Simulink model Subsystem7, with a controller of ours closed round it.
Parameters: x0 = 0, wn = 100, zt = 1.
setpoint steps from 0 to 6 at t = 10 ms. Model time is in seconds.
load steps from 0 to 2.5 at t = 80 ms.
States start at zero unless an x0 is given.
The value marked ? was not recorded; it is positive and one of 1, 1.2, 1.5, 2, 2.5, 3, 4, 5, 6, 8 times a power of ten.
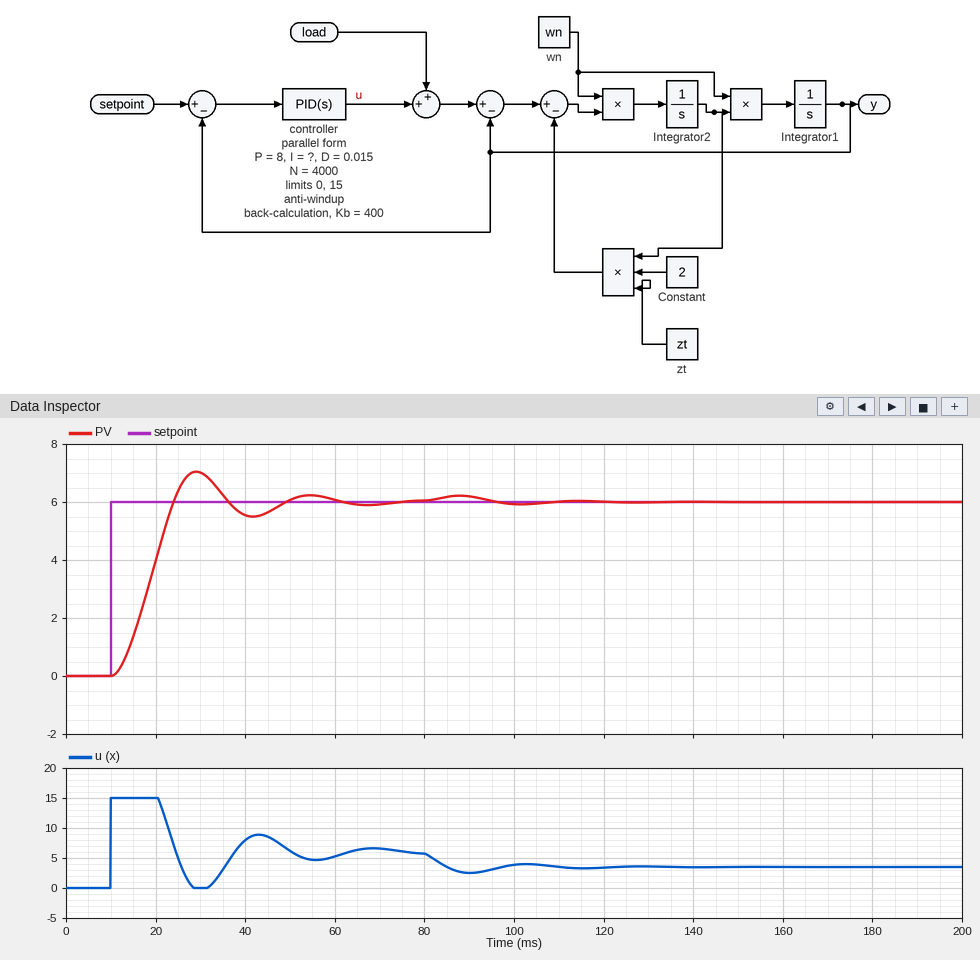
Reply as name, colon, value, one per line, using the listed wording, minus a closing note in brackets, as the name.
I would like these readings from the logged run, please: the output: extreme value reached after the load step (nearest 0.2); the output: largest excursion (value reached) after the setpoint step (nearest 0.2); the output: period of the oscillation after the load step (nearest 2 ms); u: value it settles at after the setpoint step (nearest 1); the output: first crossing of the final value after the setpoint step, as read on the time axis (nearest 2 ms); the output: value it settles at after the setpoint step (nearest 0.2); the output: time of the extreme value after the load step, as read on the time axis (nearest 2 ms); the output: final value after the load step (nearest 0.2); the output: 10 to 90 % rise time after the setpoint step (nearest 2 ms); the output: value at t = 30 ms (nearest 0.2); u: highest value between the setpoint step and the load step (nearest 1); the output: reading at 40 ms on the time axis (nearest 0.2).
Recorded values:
the output: extreme value reached after the load step: 6.2
the output: largest excursion (value reached) after the setpoint step: 7.0
the output: period of the oscillation after the load step: 26 ms
u: value it settles at after the setpoint step: 6
the output: first crossing of the final value after the setpoint step, as read on the time axis: 24 ms
the output: value it settles at after the setpoint step: 6.0
the output: time of the extreme value after the load step, as read on the time axis: 88 ms
the output: final value after the load step: 6.0
the output: 10 to 90 % rise time after the setpoint step: 10 ms
the output: value at t = 30 ms: 7.0
u: highest value between the setpoint step and the load step: 15
the output: reading at 40 ms on the time axis: 5.6
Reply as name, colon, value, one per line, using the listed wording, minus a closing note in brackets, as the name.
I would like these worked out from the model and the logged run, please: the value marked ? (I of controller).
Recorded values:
the value marked ?: 1500
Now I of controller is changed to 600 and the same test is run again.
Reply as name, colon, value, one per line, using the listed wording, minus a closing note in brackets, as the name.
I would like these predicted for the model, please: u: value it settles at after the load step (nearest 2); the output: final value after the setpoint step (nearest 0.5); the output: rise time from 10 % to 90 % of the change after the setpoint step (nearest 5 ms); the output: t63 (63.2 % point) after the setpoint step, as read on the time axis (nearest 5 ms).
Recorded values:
u: value it settles at after the load step: 4
the output: final value after the setpoint step: 6.0
the output: rise time from 10 % to 90 % of the change after the setpoint step: 20 ms
the output: t63 (63.2 % point) after the setpoint step, as read on the time axis: 20 ms
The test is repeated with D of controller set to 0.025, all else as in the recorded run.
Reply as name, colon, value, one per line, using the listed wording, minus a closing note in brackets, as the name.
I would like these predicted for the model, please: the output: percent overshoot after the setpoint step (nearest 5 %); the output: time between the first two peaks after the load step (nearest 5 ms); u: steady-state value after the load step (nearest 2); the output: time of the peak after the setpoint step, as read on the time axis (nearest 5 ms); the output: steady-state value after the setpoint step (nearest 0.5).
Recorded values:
the output: percent overshoot after the setpoint step: 20 %
the output: time between the first two peaks after the load step: 30 ms
u: steady-state value after the load step: 4
the output: time of the peak after the setpoint step, as read on the time axis: 30 ms
the output: steady-state value after the setpoint step: 6.0
